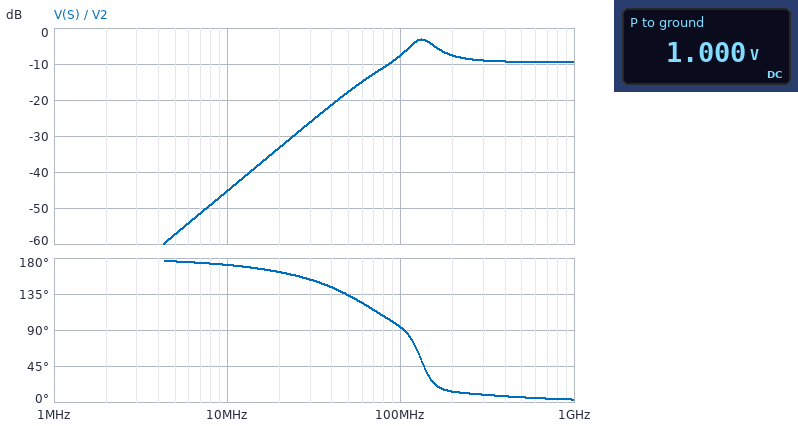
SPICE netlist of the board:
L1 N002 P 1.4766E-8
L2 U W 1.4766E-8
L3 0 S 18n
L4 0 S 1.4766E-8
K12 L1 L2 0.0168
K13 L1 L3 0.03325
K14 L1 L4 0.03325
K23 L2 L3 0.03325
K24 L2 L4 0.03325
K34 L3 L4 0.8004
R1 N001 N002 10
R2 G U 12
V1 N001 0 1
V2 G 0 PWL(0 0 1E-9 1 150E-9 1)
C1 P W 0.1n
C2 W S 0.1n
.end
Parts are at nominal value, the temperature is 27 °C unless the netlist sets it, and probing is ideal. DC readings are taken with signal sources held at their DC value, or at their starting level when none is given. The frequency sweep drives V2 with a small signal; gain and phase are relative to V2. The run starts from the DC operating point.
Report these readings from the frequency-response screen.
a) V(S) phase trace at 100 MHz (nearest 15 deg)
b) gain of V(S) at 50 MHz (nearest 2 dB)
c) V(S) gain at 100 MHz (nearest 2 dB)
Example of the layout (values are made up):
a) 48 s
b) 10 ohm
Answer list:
a) 90 deg
b) -18 dB
c) -8 dB
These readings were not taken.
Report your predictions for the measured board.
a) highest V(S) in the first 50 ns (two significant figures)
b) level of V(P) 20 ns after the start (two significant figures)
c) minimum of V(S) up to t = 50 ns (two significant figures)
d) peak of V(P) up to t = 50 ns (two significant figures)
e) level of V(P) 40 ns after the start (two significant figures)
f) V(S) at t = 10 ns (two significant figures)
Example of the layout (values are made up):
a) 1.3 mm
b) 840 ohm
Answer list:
a) 270 mV
b) 1.0 V
c) -150 mV
d) 1.3 V
e) 1.0 V
f) 23 mV
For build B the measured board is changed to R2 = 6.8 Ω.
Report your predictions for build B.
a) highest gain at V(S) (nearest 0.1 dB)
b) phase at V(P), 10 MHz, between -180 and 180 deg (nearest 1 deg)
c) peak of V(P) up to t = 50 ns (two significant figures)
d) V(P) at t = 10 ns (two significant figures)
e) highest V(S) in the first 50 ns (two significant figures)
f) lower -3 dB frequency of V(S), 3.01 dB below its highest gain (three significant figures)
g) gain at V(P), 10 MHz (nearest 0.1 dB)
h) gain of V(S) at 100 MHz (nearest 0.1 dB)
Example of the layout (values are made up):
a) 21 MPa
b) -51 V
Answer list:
a) -1.1 dB
b) 87 deg
c) 1.3 V
d) 880 mV
e) 300 mV
f) 99.2 MHz
g) -23.9 dB
h) -4.0 dB
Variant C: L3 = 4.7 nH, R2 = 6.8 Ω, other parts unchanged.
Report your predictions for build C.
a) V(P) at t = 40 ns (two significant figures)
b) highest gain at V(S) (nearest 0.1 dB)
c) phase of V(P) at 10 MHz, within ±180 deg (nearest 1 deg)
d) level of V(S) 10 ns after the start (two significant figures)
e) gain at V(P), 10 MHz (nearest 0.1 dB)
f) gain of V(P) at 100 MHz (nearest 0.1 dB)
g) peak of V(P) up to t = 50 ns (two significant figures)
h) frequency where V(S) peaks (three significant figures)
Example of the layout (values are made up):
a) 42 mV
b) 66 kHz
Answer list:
a) 1.0 V
b) -8.7 dB
c) 87 deg
d) -10 mV
e) -23.9 dB
f) -2.5 dB
g) 1.4 V
h) 182 MHz
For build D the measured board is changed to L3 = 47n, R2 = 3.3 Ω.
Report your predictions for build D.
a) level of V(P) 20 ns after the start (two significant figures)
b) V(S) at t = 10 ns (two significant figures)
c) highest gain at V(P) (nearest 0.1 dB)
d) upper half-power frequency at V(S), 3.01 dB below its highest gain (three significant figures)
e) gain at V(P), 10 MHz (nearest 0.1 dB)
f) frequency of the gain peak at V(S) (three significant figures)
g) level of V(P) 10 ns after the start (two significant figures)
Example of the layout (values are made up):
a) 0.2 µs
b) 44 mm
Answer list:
a) 990 mV
b) 90 mV
c) 0.6 dB
d) 159 MHz
e) -23.9 dB
f) 128 MHz
g) 790 mV
